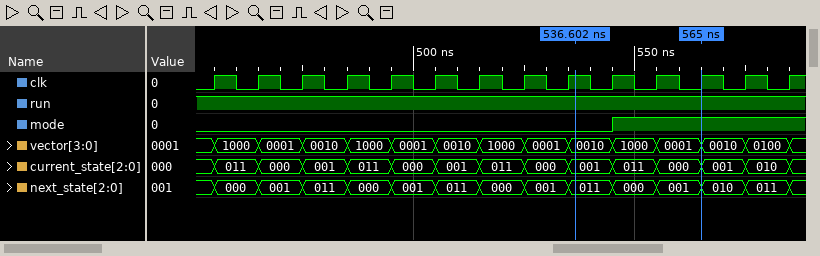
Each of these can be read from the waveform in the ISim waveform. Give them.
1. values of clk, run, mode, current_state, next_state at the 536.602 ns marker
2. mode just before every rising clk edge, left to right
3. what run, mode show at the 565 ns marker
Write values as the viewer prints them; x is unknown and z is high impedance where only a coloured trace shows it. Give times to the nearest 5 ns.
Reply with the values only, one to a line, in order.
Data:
clk=1, run=1, mode=0, current_state=001, next_state=011
0 0 0 0 0 0 0 0 0 0 1 1 1 1
run=1, mode=1
